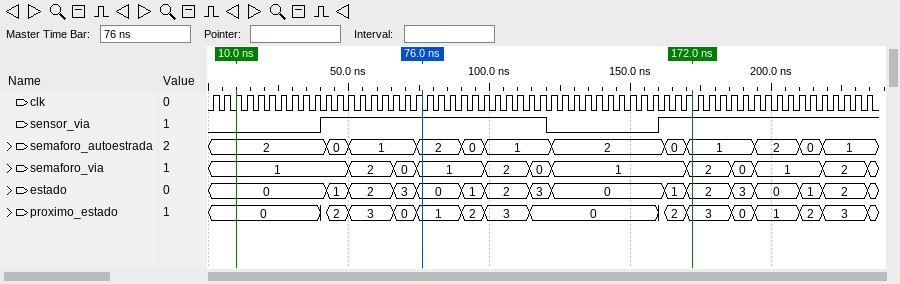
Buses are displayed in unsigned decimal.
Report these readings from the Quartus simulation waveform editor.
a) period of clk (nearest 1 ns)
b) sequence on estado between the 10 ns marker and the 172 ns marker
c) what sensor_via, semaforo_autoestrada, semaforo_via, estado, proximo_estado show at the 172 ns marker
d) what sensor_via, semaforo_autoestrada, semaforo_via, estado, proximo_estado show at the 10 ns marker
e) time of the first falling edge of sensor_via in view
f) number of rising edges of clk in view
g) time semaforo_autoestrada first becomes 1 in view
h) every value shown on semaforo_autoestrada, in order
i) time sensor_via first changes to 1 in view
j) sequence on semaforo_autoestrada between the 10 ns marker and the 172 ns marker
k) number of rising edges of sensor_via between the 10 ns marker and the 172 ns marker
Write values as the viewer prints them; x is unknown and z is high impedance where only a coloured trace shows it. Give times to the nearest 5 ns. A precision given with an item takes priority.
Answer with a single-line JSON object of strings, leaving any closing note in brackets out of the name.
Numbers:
{"period of clk": "4 ns", "sequence on estado between the 10 ns marker and the 172 ns marker": "0, 1, 2, 3, 0, 1, 2, 3, 0, 1, 2", "what sensor_via, semaforo_autoestrada, semaforo_via, estado, proximo_estado show at the 172 ns marker": "sensor_via=1, semaforo_autoestrada=1, semaforo_via=2, estado=2, proximo_estado=3", "what sensor_via, semaforo_autoestrada, semaforo_via, estado, proximo_estado show at the 10 ns marker": "sensor_via=0, semaforo_autoestrada=2, semaforo_via=1, estado=0, proximo_estado=0", "time of the first falling edge of sensor_via in view": "120 ns", "number of rising edges of clk in view": "59", "time semaforo_autoestrada first becomes 1 in view": "50 ns", "every value shown on semaforo_autoestrada, in order": "2, 0, 1, 2, 0, 1, 2, 0, 1, 2, 0, 1", "time sensor_via first changes to 1 in view": "40 ns", "sequence on semaforo_autoestrada between the 10 ns marker and the 172 ns marker": "2, 0, 1, 2, 0, 1, 2, 0, 1", "number of rising edges of sensor_via between the 10 ns marker and the 172 ns marker": "2"}
